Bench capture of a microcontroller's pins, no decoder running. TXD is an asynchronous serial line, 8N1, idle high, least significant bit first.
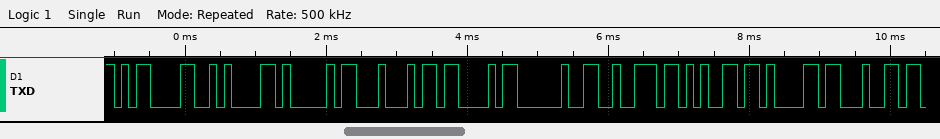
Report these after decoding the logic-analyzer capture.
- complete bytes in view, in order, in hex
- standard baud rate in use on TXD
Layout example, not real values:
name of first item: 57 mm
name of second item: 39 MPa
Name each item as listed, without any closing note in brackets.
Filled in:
complete bytes in view, in order, in hex: 0x0D 0x0A 0x41 0x44 0x43 0x20 0x72 0x65 0x61 0x64
standard baud rate in use on TXD: 9600 baud
